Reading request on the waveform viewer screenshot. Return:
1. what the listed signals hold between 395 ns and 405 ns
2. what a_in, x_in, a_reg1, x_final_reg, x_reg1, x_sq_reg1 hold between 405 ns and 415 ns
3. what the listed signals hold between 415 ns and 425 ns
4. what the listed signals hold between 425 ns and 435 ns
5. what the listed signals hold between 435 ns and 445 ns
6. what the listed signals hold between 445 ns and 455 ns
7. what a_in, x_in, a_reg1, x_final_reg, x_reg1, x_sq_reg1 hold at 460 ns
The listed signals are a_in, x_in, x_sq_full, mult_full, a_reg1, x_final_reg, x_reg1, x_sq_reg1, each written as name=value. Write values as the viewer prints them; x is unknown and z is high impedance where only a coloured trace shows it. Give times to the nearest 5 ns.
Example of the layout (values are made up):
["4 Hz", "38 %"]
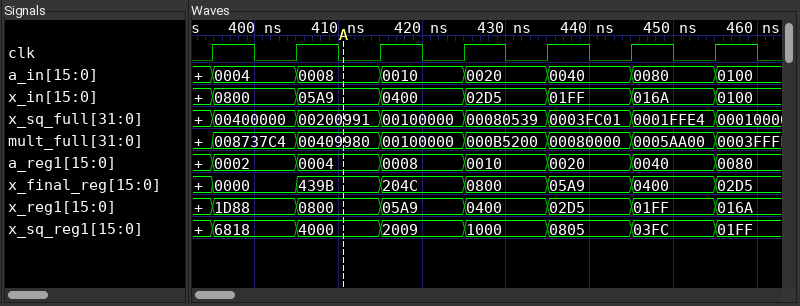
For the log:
["a_in=0004, x_in=0800, x_sq_full=00400000, mult_full=008737C4, a_reg1=0002, x_final_reg=0000, x_reg1=1D88, x_sq_reg1=6818", "a_in=0008, x_in=05A9, a_reg1=0004, x_final_reg=439B, x_reg1=0800, x_sq_reg1=4000", "a_in=0010, x_in=0400, x_sq_full=00100000, mult_full=00100000, a_reg1=0008, x_final_reg=204C, x_reg1=05A9, x_sq_reg1=2009", "a_in=0020, x_in=02D5, x_sq_full=00080539, mult_full=000B5200, a_reg1=0010, x_final_reg=0800, x_reg1=0400, x_sq_reg1=1000", "a_in=0040, x_in=01FF, x_sq_full=0003FC01, mult_full=00080000, a_reg1=0020, x_final_reg=05A9, x_reg1=02D5, x_sq_reg1=0805", "a_in=0080, x_in=016A, x_sq_full=0001FFE4, mult_full=0005AA00, a_reg1=0040, x_final_reg=0400, x_reg1=01FF, x_sq_reg1=03FC", "a_in=0100, x_in=0100, a_reg1=0080, x_final_reg=02D5, x_reg1=016A, x_sq_reg1=01FF"]
